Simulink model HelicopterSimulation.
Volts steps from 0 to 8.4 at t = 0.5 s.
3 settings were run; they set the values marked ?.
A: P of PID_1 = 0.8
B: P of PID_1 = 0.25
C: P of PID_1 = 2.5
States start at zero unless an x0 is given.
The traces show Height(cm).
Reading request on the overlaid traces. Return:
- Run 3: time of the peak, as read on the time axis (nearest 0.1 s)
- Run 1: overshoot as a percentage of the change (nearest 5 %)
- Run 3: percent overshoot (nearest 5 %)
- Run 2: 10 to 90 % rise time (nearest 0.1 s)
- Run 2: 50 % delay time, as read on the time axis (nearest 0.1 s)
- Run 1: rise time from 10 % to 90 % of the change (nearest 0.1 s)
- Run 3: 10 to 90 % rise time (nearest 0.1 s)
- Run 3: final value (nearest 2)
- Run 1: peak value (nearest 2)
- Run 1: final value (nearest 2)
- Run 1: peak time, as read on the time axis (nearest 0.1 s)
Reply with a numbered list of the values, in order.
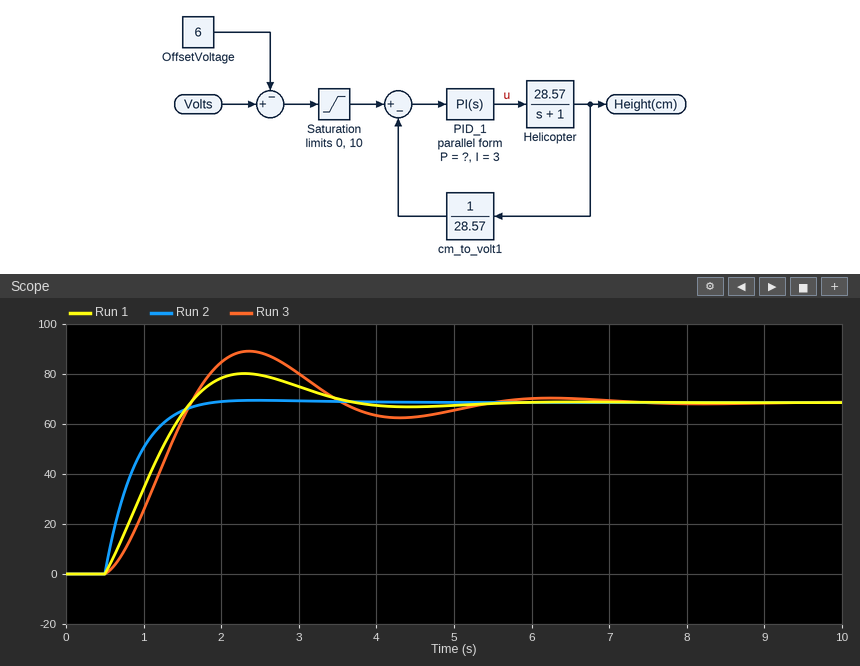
1. 2.4 s
2. 15 %
3. 30 %
4. 0.8 s
5. 0.8 s
6. 0.8 s
7. 0.8 s
8. 68
9. 80
10. 68
11. 2.3 s
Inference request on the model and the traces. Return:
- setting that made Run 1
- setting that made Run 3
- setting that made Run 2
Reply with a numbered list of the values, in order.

1. A
2. B
3. C
